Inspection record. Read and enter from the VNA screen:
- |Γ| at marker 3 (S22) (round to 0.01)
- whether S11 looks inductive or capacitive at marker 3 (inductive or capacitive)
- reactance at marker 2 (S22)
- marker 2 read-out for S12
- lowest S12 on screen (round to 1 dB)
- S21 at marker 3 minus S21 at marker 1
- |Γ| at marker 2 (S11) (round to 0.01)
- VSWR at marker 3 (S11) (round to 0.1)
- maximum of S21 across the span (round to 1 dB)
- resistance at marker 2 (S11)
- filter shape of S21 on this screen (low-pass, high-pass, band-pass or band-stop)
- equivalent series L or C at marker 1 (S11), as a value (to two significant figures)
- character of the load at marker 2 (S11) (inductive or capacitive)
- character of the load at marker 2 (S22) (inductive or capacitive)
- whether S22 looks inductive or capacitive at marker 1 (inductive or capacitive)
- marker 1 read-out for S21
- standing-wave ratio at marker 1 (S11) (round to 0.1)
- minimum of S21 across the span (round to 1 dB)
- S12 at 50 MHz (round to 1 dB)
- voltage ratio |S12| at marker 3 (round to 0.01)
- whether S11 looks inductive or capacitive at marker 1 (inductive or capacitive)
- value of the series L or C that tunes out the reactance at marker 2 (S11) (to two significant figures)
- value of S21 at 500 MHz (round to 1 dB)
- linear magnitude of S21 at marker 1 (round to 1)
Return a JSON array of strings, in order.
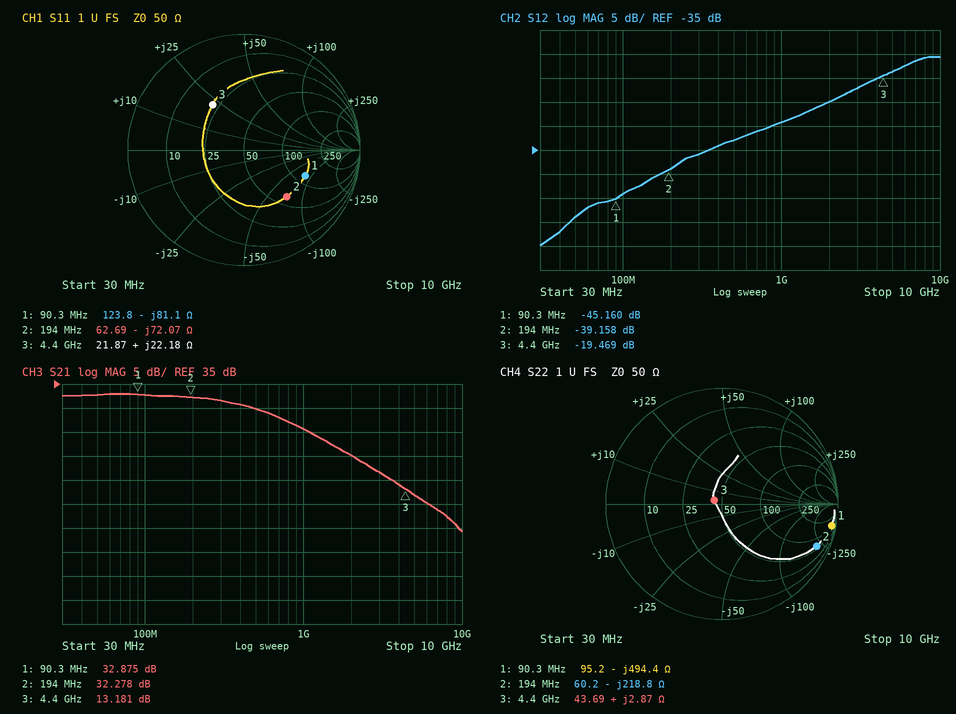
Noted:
["0.07", "inductive", "-218.8 Ω", "-39.158 dB", "-55 dB", "-19.694 dB", "0.55", "2.8", "33 dB", "62.69 Ω", "low-pass", "22 pF", "capacitive", "capacitive", "capacitive", "32.875 dB", "3.7", "4 dB", "-49 dB", "0.11", "capacitive", "59 nH", "30 dB", "44"]
